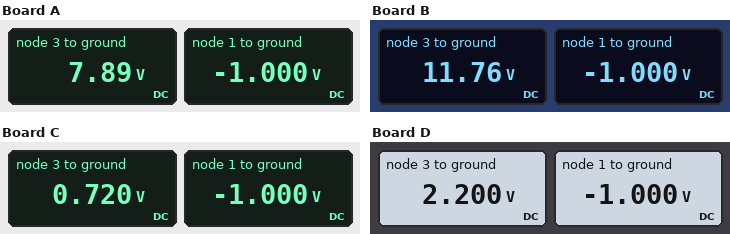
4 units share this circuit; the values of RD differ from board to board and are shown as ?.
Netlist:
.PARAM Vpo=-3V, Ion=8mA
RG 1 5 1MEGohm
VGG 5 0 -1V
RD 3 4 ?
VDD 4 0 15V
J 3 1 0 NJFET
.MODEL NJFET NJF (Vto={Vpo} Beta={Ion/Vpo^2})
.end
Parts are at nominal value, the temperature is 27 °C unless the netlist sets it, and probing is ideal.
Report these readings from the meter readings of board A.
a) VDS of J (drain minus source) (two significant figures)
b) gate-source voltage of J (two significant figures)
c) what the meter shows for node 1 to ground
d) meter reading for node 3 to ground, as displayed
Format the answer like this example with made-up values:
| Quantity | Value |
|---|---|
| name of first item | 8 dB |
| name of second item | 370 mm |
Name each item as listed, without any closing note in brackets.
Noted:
| Quantity | Value |
|---|---|
| VDS of J (drain minus source) | 7.9 V |
| gate-source voltage of J | -1.0 V |
| what the meter shows for node 1 to ground | -1.000 V |
| meter reading for node 3 to ground, as displayed | 7.89 V |
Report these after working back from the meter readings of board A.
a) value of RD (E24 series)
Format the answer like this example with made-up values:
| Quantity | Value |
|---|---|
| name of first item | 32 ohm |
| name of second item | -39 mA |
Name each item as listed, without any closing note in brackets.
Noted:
| Quantity | Value |
|---|---|
| value of RD | 2 kΩ |
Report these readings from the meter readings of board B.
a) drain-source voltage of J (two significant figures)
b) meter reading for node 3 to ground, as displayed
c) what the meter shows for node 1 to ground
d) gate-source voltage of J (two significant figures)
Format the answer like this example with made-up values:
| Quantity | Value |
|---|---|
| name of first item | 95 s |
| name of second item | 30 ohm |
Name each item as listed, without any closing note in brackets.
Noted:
| Quantity | Value |
|---|---|
| drain-source voltage of J | 12 V |
| meter reading for node 3 to ground, as displayed | 11.76 V |
| what the meter shows for node 1 to ground | -1.000 V |
| gate-source voltage of J | -1.0 V |
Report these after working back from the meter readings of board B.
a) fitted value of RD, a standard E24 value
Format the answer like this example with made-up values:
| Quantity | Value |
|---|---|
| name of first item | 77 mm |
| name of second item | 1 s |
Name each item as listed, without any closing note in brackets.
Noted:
| Quantity | Value |
|---|---|
| fitted value of RD, a standard E24 value | 910 Ω |
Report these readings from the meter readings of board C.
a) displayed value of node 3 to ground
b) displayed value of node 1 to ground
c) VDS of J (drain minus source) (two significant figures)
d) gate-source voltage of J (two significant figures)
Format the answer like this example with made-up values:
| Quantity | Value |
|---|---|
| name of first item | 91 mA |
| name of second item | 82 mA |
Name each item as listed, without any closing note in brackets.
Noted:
| Quantity | Value |
|---|---|
| displayed value of node 3 to ground | 0.720 V |
| displayed value of node 1 to ground | -1.000 V |
| VDS of J (drain minus source) | 720 mV |
| gate-source voltage of J | -1.0 V |
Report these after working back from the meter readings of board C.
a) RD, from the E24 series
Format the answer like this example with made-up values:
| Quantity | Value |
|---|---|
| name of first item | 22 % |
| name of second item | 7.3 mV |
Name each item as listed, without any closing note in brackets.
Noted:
| Quantity | Value |
|---|---|
| RD, from the E24 series | 6.8 kΩ |
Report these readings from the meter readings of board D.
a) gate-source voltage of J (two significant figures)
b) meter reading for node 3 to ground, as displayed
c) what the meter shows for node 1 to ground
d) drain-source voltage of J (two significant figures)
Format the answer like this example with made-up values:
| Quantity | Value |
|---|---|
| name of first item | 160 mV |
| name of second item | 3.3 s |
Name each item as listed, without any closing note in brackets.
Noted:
| Quantity | Value |
|---|---|
| gate-source voltage of J | -1.0 V |
| meter reading for node 3 to ground, as displayed | 2.200 V |
| what the meter shows for node 1 to ground | -1.000 V |
| drain-source voltage of J | 2.2 V |
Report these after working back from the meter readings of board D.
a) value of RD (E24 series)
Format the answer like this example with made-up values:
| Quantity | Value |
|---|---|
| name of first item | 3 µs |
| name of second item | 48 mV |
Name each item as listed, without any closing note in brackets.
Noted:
| Quantity | Value |
|---|---|
| value of RD | 3.6 kΩ |
